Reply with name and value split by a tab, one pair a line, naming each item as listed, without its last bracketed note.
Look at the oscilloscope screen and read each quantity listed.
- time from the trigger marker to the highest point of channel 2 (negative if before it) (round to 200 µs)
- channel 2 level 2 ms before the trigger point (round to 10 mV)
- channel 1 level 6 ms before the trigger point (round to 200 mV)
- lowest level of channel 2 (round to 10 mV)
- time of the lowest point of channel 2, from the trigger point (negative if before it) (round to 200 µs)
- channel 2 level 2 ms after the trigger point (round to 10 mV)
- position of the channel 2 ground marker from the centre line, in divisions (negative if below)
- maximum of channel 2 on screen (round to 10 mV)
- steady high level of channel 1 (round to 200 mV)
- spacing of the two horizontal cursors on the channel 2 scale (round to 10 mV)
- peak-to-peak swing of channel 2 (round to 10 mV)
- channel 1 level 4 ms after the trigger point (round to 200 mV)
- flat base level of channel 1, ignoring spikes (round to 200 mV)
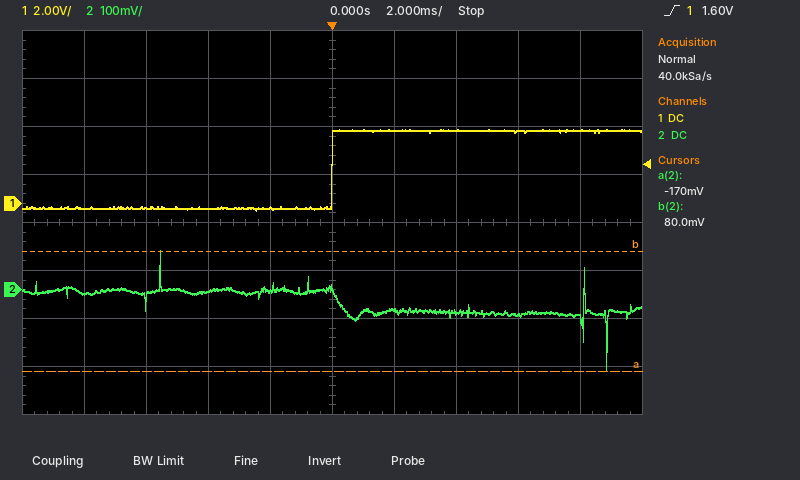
time from the trigger marker to the highest point of channel 2 (negative if before it)	-5.6 ms
channel 2 level 2 ms before the trigger point	0 mV
channel 1 level 6 ms before the trigger point	-200 mV
lowest level of channel 2	-170 mV
time of the lowest point of channel 2, from the trigger point (negative if before it)	+8.8 ms
channel 2 level 2 ms after the trigger point	-40 mV
position of the channel 2 ground marker from the centre line, in divisions	-1.4 div
maximum of channel 2 on screen	80 mV
steady high level of channel 1	3.0 V
spacing of the two horizontal cursors on the channel 2 scale	250 mV
peak-to-peak swing of channel 2	250 mV
channel 1 level 4 ms after the trigger point	3.0 V
flat base level of channel 1, ignoring spikes	-200 mV
